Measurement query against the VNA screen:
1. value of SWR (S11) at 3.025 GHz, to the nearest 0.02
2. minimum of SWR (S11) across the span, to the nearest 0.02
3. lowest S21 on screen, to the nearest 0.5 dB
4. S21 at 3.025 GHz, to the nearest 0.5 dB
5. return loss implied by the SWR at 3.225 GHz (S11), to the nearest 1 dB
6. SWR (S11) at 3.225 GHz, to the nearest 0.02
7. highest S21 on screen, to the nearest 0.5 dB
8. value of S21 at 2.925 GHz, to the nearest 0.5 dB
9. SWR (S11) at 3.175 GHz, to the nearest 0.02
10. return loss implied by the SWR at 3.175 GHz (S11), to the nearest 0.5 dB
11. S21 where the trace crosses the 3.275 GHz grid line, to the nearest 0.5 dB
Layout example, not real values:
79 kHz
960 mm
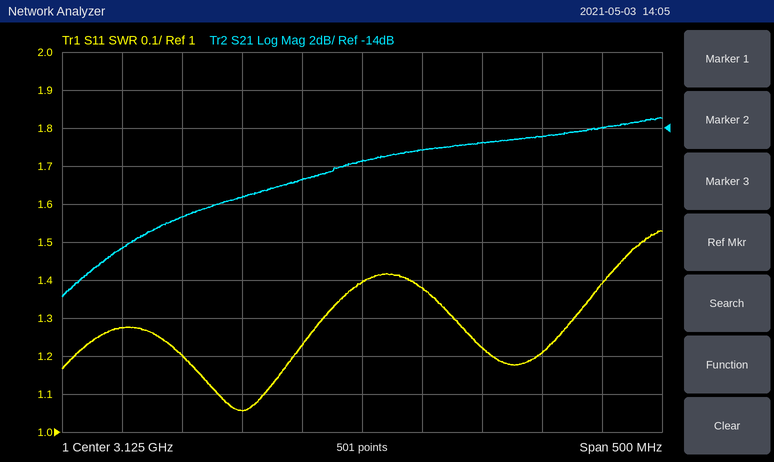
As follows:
1.06
1.06
-23.0 dB
-17.5 dB
20 dB
1.22
-13.5 dB
-20.5 dB
1.38
16.0 dB
-14.5 dB
